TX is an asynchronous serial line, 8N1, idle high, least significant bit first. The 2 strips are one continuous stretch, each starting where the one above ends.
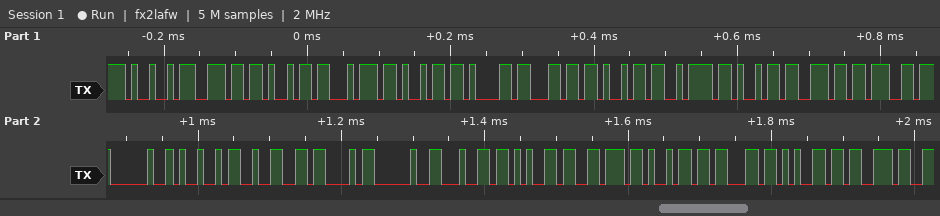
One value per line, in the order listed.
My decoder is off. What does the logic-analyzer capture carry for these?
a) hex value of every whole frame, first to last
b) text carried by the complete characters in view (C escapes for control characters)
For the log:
49 6E 69 74 69 61 6C 69 7A 69 6E 67 20 49 32 43 20 64 65 76 69 63 65 73
"Initializing I2C devices"
